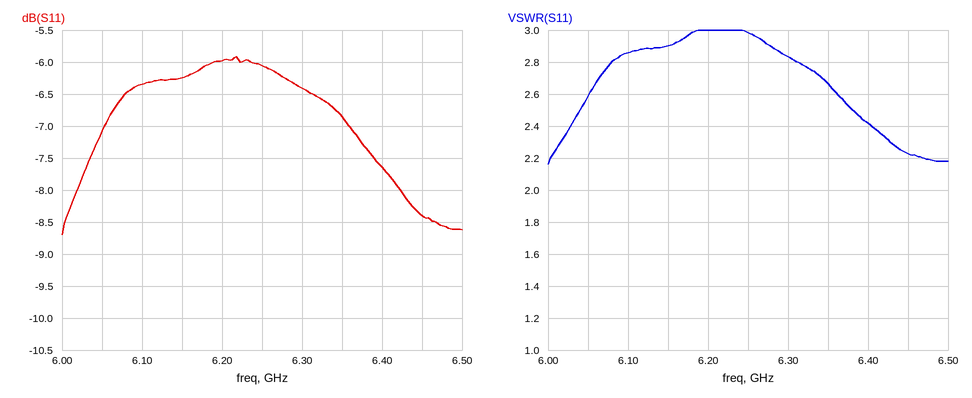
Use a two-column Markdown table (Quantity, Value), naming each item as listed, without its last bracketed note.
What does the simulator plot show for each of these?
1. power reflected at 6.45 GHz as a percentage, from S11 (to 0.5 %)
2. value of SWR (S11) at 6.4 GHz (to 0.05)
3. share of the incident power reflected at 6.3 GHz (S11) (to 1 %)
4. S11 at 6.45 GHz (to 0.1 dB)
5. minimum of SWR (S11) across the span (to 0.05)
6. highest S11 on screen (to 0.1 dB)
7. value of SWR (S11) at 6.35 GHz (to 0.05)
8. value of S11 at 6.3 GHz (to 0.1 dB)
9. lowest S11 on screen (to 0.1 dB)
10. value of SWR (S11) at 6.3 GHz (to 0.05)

| Quantity | Value |
|---|---|
| power reflected at 6.45 GHz as a percentage, from S11 | 14.5 % |
| value of SWR (S11) at 6.4 GHz | 2.40 |
| share of the incident power reflected at 6.3 GHz (S11) | 23 % |
| S11 at 6.45 GHz | -8.4 dB |
| minimum of SWR (S11) across the span | 2.15 |
| highest S11 on screen | -5.9 dB |
| value of SWR (S11) at 6.35 GHz | 2.65 |
| value of S11 at 6.3 GHz | -6.4 dB |
| lowest S11 on screen | -8.7 dB |
| value of SWR (S11) at 6.3 GHz | 2.85 |
